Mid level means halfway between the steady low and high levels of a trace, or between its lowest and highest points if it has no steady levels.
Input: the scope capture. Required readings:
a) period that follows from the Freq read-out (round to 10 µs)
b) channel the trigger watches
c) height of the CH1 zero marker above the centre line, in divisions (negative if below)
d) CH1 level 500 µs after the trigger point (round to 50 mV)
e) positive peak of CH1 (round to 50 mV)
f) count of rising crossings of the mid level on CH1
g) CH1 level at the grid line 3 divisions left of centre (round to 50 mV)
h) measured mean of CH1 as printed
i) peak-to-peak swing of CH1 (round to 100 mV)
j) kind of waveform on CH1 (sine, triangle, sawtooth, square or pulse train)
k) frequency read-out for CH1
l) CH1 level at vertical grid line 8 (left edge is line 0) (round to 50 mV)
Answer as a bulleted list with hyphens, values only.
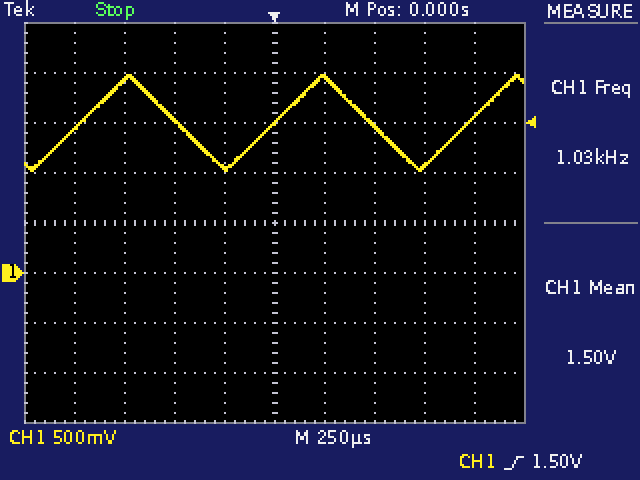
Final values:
- 970 µs
- CH1
- -1.0 div
- 1.45 V
- 2.00 V
- 3
- 1.95 V
- 1.50 V
- 1.00 V
- triangle
- 1.03 kHz
- 1.05 V
